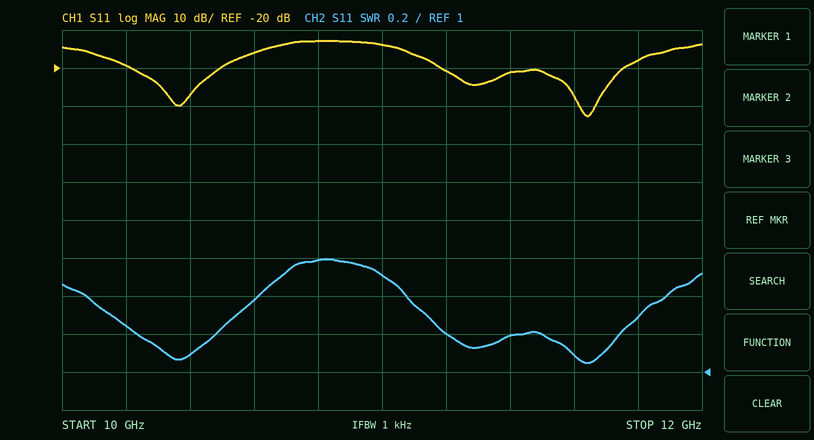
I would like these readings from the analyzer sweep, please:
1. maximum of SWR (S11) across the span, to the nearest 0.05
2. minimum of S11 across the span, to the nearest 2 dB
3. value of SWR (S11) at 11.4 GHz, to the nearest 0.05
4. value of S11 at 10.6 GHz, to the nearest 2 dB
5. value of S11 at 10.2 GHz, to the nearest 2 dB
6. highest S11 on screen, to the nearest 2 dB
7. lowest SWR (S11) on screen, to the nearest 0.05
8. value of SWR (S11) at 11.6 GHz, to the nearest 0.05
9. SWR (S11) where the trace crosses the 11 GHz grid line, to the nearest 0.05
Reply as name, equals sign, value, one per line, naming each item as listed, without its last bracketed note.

maximum of SWR (S11) across the span, to the nearest 0.05 = 1.60
minimum of S11 across the span, to the nearest 2 dB = -32 dB
value of SWR (S11) at 11.4 GHz, to the nearest 0.05 = 1.20
value of S11 at 10.6 GHz, to the nearest 2 dB = -16 dB
value of S11 at 10.2 GHz, to the nearest 2 dB = -20 dB
highest S11 on screen, to the nearest 2 dB = -12 dB
lowest SWR (S11) on screen, to the nearest 0.05 = 1.05
value of SWR (S11) at 11.6 GHz, to the nearest 0.05 = 1.10
SWR (S11) where the trace crosses the 11 GHz grid line, to the nearest 0.05 = 1.50
